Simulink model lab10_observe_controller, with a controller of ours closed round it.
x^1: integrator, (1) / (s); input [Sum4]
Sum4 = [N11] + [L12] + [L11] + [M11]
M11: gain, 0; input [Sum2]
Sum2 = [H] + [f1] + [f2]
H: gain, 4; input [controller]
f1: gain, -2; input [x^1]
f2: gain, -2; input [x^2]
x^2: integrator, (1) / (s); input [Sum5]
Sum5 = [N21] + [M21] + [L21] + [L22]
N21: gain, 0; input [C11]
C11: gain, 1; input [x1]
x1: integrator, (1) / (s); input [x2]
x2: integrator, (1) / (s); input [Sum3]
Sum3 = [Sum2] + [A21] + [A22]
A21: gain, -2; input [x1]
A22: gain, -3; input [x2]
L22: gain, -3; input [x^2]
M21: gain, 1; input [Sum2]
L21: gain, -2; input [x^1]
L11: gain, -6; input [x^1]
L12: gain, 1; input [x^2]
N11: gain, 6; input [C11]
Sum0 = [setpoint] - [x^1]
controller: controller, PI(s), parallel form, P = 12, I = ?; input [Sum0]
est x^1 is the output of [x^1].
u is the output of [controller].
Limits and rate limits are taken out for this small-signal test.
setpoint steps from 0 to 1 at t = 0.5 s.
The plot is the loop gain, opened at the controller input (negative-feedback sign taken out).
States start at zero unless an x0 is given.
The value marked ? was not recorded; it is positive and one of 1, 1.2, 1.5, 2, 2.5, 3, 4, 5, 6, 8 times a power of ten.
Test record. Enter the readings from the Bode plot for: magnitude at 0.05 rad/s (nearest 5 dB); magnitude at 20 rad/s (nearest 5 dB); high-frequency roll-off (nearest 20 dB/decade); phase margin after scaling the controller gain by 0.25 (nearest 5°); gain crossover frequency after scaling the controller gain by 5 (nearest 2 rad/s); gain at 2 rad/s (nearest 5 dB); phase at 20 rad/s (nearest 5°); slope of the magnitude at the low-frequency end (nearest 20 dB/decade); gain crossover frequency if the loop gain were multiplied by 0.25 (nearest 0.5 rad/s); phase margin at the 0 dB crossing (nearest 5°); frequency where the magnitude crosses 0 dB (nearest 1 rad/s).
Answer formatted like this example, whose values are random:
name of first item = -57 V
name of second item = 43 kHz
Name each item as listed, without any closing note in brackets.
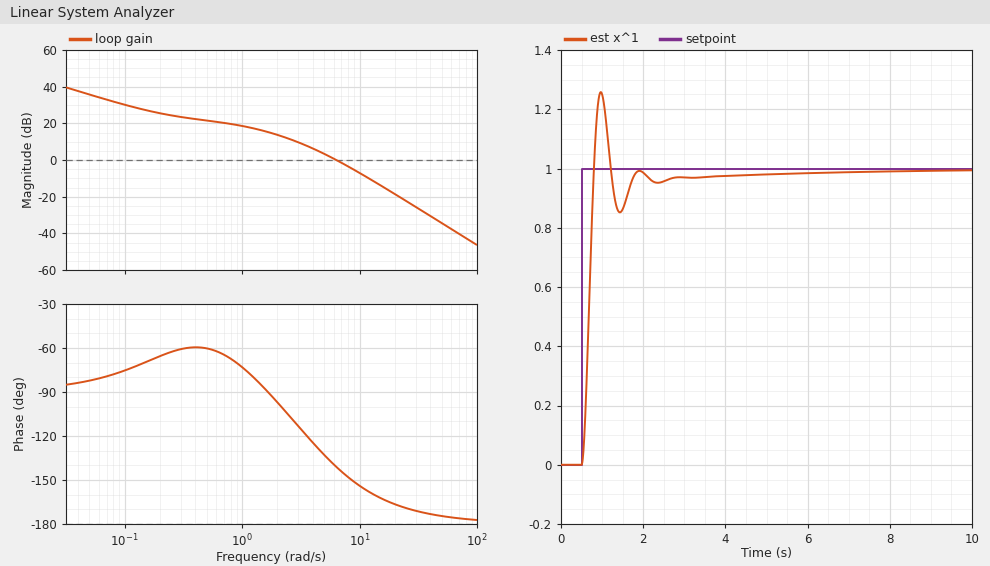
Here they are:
magnitude at 0.05 rad/s = 35 dB
magnitude at 20 rad/s = -20 dB
high-frequency roll-off = -40 dB/decade
phase margin after scaling the controller gain by 0.25 = 75°
gain crossover frequency after scaling the controller gain by 5 = 16 rad/s
gain at 2 rad/s = 15 dB
phase at 20 rad/s = -165°
slope of the magnitude at the low-frequency end = -20 dB/decade
gain crossover frequency if the loop gain were multiplied by 0.25 = 2.5 rad/s
phase margin at the 0 dB crossing = 40°
frequency where the magnitude crosses 0 dB = 6 rad/s
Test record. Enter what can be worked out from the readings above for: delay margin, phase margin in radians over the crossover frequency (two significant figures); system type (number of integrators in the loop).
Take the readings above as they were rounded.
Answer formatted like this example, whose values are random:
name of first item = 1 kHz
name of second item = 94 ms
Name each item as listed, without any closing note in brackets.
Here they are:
delay margin, phase margin in radians over the crossover frequency = 0.12 s
system type = 1
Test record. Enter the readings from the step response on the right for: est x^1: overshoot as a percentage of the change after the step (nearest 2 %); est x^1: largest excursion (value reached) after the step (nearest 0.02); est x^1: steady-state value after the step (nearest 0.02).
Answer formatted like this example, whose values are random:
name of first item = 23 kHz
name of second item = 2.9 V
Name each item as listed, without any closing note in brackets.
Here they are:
est x^1: overshoot as a percentage of the change after the step = 26 %
est x^1: largest excursion (value reached) after the step = 1.26
est x^1: steady-state value after the step = 1.00
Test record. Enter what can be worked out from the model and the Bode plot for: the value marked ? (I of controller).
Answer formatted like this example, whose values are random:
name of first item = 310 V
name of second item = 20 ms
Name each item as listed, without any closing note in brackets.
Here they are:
the value marked ? = 3
